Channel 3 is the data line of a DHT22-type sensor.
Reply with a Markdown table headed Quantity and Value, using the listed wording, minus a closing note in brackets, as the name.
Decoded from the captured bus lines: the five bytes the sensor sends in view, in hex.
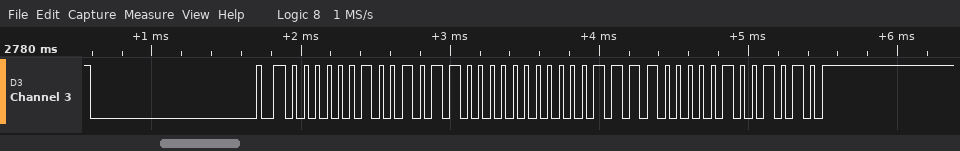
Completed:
| Quantity | Value |
|---|---|
| the five bytes the sensor sends in view, in hex | 02, 58, 00, F0, 4A |
